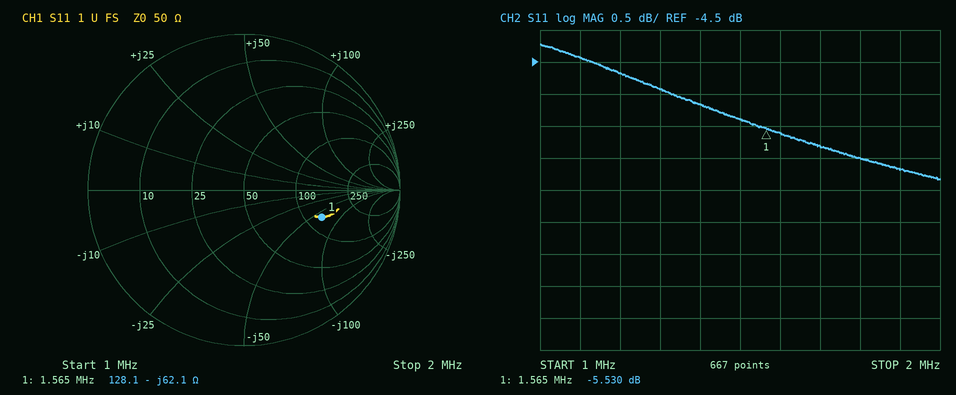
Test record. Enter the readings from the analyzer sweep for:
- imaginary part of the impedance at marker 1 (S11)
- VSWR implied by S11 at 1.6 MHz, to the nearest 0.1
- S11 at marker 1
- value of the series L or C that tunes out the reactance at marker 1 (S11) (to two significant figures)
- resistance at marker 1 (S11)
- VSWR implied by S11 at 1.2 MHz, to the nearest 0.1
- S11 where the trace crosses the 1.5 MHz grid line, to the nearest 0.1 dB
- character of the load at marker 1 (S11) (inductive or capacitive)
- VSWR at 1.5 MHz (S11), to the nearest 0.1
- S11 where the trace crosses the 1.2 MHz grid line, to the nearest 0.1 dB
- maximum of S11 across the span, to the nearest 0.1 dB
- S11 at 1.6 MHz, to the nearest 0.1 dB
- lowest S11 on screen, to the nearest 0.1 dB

-62.1 Ω
3.2
-5.530 dB
6.3 µH
128.1 Ω
3.8
-5.4 dB
capacitive
3.3
-4.7 dB
-4.2 dB
-5.6 dB
-6.3 dB
